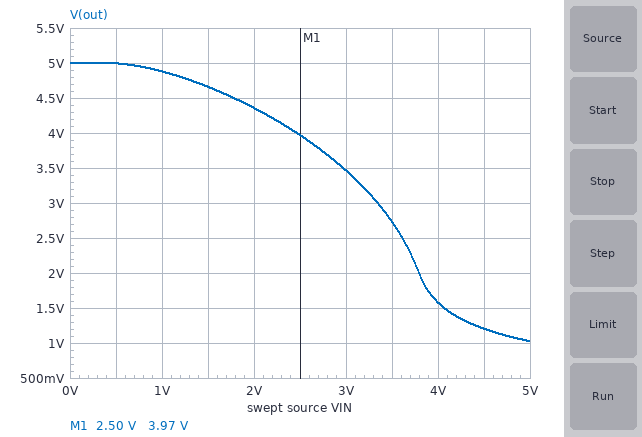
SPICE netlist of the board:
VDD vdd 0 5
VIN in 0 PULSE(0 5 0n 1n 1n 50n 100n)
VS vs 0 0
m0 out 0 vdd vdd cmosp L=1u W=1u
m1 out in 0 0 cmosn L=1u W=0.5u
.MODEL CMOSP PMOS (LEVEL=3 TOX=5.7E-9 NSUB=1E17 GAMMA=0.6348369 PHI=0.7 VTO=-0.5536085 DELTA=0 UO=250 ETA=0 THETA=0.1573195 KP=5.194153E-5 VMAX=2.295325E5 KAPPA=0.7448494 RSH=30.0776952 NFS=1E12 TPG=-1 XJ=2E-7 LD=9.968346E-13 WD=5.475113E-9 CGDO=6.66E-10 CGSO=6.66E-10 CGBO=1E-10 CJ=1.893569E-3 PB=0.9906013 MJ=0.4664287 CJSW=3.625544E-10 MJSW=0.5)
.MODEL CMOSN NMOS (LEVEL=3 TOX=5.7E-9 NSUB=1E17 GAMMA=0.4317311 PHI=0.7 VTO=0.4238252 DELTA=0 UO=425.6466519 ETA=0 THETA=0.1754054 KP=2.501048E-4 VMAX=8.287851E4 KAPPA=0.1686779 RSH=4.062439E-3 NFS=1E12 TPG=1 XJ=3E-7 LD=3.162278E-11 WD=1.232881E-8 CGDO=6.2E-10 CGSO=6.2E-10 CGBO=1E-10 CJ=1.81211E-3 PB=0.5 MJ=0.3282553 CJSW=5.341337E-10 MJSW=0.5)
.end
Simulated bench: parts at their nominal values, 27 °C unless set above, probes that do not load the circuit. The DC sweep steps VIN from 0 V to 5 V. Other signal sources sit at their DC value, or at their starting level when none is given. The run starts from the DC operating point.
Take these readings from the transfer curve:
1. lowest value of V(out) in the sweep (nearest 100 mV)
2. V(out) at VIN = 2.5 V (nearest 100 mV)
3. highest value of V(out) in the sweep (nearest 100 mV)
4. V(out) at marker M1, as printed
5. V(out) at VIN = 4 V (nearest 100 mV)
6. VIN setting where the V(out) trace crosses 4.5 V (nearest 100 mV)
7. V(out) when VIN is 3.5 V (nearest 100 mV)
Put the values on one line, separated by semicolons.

1.0 V; 4.0 V; 5.0 V; 3.97 V; 1.6 V; 1.8 V; 2.7 V
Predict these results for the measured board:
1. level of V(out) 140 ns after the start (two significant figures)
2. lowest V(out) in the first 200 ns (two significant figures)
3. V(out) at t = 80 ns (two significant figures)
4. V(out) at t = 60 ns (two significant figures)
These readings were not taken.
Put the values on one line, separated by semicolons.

1.0 V; 1.0 V; 5.0 V; 5.0 V
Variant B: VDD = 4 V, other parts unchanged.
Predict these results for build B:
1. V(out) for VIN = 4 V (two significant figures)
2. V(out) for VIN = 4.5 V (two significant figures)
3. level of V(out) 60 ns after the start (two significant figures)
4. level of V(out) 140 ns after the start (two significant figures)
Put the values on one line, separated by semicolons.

770 mV; 670 mV; 4.0 V; 600 mV
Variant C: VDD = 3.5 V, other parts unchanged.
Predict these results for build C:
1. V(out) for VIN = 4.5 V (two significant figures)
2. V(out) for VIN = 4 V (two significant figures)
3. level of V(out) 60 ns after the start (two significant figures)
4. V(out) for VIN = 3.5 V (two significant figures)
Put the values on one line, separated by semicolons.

490 mV; 550 mV; 3.5 V; 650 mV
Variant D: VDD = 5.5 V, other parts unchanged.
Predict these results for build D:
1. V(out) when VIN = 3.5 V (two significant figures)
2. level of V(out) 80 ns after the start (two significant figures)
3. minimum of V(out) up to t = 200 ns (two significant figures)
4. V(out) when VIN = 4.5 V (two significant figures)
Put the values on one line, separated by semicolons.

3.6 V; 5.5 V; 1.3 V; 1.7 V
